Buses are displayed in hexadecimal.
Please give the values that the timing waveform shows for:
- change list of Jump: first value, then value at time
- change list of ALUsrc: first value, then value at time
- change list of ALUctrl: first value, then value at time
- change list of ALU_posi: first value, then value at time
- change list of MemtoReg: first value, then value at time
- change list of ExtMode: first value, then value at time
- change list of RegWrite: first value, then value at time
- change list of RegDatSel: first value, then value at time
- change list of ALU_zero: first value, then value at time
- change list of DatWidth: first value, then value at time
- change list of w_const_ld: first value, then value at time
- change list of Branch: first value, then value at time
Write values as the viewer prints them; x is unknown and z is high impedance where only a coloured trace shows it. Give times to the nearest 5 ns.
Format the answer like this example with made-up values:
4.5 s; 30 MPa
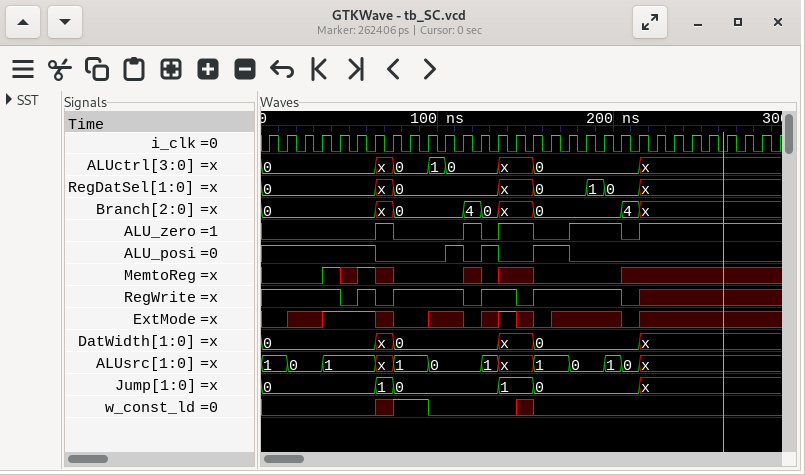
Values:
0, 1 at 65 ns, 0 at 75 ns, 1 at 135 ns, 0 at 155 ns, x at 215 ns; 1, 0 at 15 ns, 1 at 35 ns, x at 65 ns, 1 at 75 ns, 0 at 95 ns, 1 at 125 ns, x at 135 ns, 1 at 155 ns, 0 at 175 ns, 1 at 195 ns, 0 at 205 ns, x at 215 ns; 0, x at 65 ns, 0 at 75 ns, 1 at 95 ns, 0 at 105 ns, x at 135 ns, 0 at 155 ns, x at 215 ns; 1, 0 at 65 ns, 1 at 105 ns, 0 at 115 ns, 1 at 125 ns, 0 at 135 ns, 1 at 155 ns, 0 at 175 ns; 0, 1 at 35 ns, x at 45 ns, 1 at 55 ns, x at 65 ns, 0 at 75 ns, x at 115 ns, 0 at 125 ns, x at 135 ns, 0 at 155 ns, x at 205 ns; 0, x at 15 ns, 1 at 35 ns, x at 65 ns, 0 at 75 ns, x at 95 ns, 0 at 115 ns, x at 125 ns, 1 at 135 ns, x at 145 ns, 0 at 155 ns, x at 165 ns, 0 at 205 ns, x at 215 ns; 1, 0 at 45 ns, 1 at 55 ns, 0 at 65 ns, 1 at 75 ns, 0 at 115 ns, 1 at 125 ns, 0 at 145 ns, 1 at 155 ns, 0 at 205 ns, x at 215 ns; 0, x at 65 ns, 0 at 75 ns, x at 135 ns, 0 at 155 ns, 1 at 185 ns, 0 at 195 ns, x at 215 ns; 0, 1 at 65 ns, 0 at 75 ns, 1 at 115 ns, 0 at 125 ns, 1 at 135 ns, 0 at 155 ns, 1 at 175 ns, 0 at 205 ns, 1 at 215 ns; 0, x at 65 ns, 0 at 75 ns, x at 135 ns, 0 at 155 ns, x at 215 ns; 0, x at 65 ns, 1 at 75 ns, 0 at 95 ns, x at 145 ns, 0 at 155 ns; 0, x at 65 ns, 0 at 75 ns, 4 at 115 ns, 0 at 125 ns, x at 135 ns, 0 at 155 ns, 4 at 205 ns, x at 215 ns
